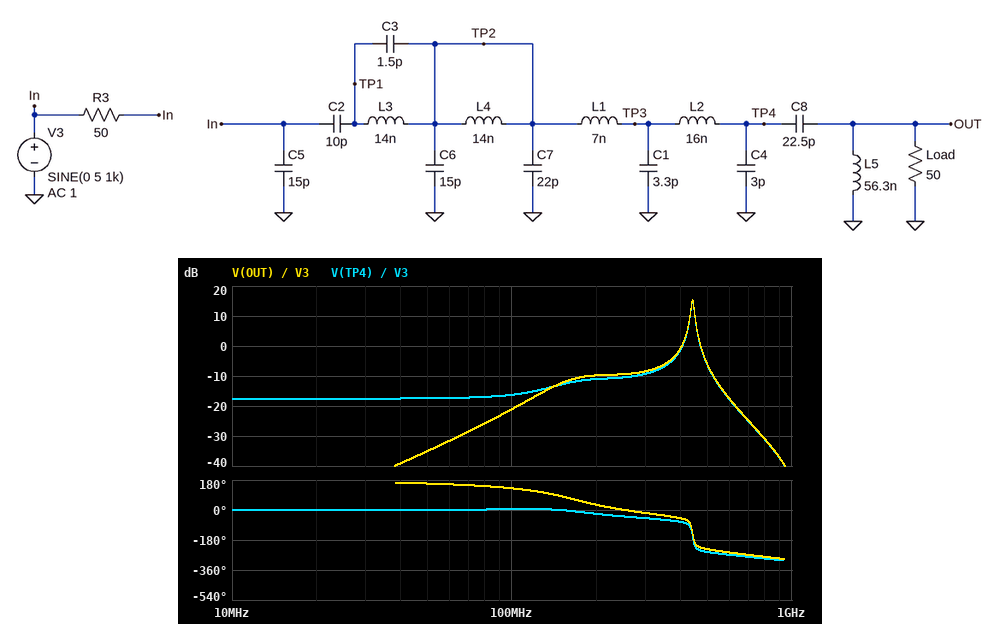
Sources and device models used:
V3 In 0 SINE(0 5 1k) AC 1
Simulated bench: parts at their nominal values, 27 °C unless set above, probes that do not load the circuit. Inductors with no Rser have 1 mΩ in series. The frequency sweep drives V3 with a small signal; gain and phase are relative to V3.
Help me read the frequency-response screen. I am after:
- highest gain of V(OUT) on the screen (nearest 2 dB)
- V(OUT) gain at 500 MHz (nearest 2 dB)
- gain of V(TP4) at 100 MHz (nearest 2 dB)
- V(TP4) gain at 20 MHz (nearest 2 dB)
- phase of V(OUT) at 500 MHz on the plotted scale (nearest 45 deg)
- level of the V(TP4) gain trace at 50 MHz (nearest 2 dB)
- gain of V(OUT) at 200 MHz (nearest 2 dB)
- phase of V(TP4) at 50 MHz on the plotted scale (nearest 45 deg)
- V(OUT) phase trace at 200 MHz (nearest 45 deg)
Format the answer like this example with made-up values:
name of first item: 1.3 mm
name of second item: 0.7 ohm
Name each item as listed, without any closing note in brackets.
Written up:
highest gain of V(OUT) on the screen: 16 dB
V(OUT) gain at 500 MHz: -6 dB
gain of V(TP4) at 100 MHz: -16 dB
V(TP4) gain at 20 MHz: -18 dB
phase of V(OUT) at 500 MHz on the plotted scale: -225 deg
level of the V(TP4) gain trace at 50 MHz: -18 dB
gain of V(OUT) at 200 MHz: -10 dB
phase of V(TP4) at 50 MHz on the plotted scale: 0 deg
V(OUT) phase trace at 200 MHz: 45 deg
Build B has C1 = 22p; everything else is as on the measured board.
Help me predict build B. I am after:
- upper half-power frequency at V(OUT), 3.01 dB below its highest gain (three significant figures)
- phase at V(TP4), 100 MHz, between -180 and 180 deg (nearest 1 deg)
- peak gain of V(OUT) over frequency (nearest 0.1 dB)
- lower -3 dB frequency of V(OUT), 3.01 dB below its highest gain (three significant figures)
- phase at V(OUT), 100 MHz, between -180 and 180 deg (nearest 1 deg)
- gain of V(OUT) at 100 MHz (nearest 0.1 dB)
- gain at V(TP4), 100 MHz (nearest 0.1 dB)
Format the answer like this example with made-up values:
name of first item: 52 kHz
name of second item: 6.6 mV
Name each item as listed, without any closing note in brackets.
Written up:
upper half-power frequency at V(OUT), 3.01 dB below its highest gain: 429 MHz
phase at V(TP4), 100 MHz, between -180 and 180 deg: 3 deg
peak gain of V(OUT) over frequency: 10.6 dB
lower -3 dB frequency of V(OUT), 3.01 dB below its highest gain: 397 MHz
phase at V(OUT), 100 MHz, between -180 and 180 deg: 129 deg
gain of V(OUT) at 100 MHz: -22.5 dB
gain at V(TP4), 100 MHz: -17.7 dB
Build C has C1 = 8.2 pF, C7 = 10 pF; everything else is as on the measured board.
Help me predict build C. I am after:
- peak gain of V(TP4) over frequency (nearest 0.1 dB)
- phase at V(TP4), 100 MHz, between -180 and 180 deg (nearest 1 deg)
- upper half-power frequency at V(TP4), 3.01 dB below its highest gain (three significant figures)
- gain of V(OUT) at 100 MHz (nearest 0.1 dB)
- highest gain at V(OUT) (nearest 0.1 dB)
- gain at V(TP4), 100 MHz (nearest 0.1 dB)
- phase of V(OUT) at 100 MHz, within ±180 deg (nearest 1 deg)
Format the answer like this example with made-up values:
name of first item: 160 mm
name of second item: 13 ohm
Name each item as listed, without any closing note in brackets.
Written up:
peak gain of V(TP4) over frequency: 10.9 dB
phase at V(TP4), 100 MHz, between -180 and 180 deg: 6 deg
upper half-power frequency at V(TP4), 3.01 dB below its highest gain: 465 MHz
gain of V(OUT) at 100 MHz: -20.4 dB
highest gain at V(OUT): 11.3 dB
gain at V(TP4), 100 MHz: -15.6 dB
phase of V(OUT) at 100 MHz, within ±180 deg: 131 deg
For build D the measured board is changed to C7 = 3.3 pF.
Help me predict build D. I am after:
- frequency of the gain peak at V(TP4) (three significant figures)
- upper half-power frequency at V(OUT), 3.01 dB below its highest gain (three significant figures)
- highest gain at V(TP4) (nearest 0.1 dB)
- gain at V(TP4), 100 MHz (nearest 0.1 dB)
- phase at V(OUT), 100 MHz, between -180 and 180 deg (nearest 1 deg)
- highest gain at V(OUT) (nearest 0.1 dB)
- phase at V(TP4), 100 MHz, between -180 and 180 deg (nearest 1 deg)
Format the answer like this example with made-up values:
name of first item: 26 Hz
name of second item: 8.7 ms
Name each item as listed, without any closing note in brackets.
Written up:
frequency of the gain peak at V(TP4): 482 MHz
upper half-power frequency at V(OUT), 3.01 dB below its highest gain: 499 MHz
highest gain at V(TP4): 9.6 dB
gain at V(TP4), 100 MHz: -14.5 dB
phase at V(OUT), 100 MHz, between -180 and 180 deg: 133 deg
highest gain at V(OUT): 10.0 dB
phase at V(TP4), 100 MHz, between -180 and 180 deg: 8 deg
